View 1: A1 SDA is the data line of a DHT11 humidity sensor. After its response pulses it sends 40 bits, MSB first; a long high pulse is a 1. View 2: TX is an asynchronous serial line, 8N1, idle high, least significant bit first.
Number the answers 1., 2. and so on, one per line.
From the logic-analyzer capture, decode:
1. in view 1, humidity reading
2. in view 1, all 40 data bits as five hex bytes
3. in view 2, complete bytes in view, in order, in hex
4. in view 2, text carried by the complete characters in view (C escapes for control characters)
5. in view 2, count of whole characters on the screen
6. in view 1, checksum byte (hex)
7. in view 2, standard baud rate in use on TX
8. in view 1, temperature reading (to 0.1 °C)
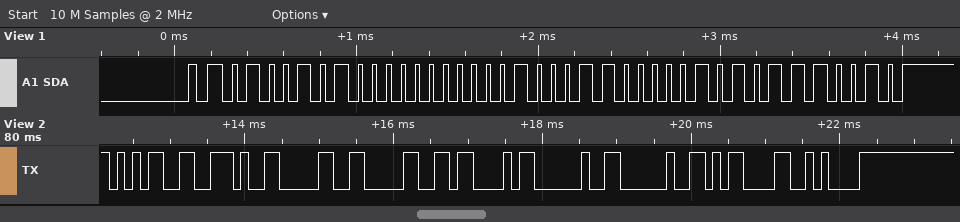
1. 74 %
2. 4A 00 23 05 72
3. 35 2E 30 30 43 20 20 0D 0A
4. "5.00C  \r\n"
5. 9
6. 0x72
7. 9600 baud
8. 35.5 °C
